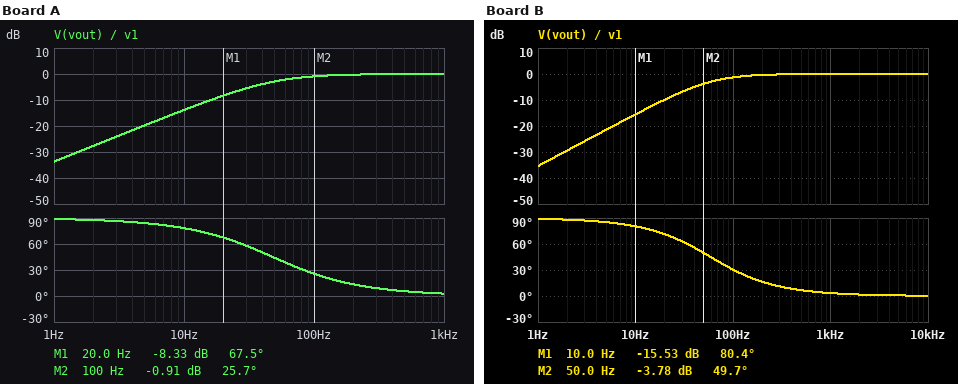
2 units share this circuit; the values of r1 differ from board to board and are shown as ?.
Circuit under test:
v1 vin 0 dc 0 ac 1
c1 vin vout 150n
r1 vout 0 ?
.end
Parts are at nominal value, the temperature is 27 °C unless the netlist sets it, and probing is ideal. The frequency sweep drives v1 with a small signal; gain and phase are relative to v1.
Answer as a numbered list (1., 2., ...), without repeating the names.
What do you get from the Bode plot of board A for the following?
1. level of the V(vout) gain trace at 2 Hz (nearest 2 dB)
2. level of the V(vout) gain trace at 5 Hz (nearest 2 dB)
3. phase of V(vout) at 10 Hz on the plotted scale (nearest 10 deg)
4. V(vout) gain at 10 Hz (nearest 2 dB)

1. -28 dB
2. -20 dB
3. 80 deg
4. -14 dB
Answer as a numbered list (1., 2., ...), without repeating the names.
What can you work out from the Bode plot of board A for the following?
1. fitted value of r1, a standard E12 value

1. 22 kΩ
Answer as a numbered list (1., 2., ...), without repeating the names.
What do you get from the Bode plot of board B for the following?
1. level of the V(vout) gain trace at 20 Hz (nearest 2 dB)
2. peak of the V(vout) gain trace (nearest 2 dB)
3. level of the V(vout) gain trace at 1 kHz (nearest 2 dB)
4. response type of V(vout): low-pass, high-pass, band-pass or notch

1. -10 dB
2. 0 dB
3. 0 dB
4. high-pass
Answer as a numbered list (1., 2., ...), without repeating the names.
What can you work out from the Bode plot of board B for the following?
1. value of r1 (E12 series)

1. 18 kΩ
